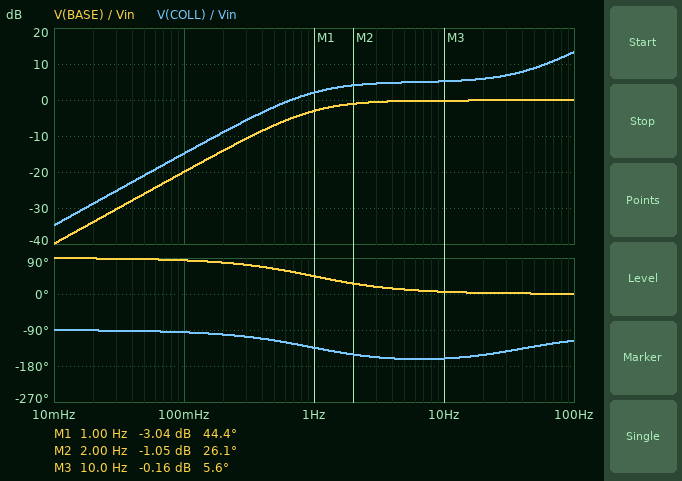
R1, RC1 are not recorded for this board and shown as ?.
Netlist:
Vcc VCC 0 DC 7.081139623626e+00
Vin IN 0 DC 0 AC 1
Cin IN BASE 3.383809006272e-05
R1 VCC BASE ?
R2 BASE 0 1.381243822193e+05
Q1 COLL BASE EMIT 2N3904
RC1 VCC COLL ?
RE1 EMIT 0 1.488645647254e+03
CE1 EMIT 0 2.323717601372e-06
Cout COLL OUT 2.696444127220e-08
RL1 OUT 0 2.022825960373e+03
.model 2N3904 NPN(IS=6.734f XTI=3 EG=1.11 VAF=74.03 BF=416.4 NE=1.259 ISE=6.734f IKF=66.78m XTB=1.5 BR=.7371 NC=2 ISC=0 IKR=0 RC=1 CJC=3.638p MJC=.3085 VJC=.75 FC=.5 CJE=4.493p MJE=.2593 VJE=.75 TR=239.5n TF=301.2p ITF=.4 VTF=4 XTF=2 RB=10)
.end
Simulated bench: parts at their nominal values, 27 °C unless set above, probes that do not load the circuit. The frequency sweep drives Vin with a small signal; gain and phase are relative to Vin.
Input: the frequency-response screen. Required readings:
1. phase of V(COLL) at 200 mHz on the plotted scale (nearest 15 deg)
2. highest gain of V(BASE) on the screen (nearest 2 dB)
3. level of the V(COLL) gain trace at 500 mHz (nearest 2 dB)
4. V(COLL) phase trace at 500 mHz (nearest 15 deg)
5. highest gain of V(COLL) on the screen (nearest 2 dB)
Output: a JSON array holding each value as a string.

["-105 deg", "0 dB", "-2 dB", "-120 deg", "14 dB"]
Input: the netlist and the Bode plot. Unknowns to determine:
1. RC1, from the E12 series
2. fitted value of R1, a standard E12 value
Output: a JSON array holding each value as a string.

["3.9 kΩ", "150 kΩ"]
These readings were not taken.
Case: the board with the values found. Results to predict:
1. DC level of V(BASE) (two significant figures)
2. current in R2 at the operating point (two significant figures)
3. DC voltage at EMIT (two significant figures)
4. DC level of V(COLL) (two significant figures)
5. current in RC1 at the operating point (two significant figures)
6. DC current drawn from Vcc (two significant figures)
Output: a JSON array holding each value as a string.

["2.6 V", "19 µA", "1.9 V", "2.1 V", "1.3 mA", "1.3 mA"]
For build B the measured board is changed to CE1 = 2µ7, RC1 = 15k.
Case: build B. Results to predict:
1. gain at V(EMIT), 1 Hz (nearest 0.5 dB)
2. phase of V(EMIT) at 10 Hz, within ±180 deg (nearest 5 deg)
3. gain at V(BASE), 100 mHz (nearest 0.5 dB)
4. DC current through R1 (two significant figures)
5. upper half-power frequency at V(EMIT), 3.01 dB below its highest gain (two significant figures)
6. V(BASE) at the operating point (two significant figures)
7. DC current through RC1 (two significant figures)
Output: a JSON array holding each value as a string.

["-11.0 dB", "15 deg", "-30.0 dB", "38 µA", "650 Hz", "1.3 V", "420 µA"]
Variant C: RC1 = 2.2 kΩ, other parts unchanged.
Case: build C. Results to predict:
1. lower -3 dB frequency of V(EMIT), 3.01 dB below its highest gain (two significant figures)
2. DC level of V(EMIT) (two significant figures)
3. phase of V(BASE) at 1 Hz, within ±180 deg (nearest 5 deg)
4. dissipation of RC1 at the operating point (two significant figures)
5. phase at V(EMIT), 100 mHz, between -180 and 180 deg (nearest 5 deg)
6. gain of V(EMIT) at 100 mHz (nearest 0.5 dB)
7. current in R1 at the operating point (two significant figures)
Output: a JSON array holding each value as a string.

["86 mHz", "2.0 V", "5 deg", "4.0 mW", "40 deg", "-2.5 dB", "29 µA"]
